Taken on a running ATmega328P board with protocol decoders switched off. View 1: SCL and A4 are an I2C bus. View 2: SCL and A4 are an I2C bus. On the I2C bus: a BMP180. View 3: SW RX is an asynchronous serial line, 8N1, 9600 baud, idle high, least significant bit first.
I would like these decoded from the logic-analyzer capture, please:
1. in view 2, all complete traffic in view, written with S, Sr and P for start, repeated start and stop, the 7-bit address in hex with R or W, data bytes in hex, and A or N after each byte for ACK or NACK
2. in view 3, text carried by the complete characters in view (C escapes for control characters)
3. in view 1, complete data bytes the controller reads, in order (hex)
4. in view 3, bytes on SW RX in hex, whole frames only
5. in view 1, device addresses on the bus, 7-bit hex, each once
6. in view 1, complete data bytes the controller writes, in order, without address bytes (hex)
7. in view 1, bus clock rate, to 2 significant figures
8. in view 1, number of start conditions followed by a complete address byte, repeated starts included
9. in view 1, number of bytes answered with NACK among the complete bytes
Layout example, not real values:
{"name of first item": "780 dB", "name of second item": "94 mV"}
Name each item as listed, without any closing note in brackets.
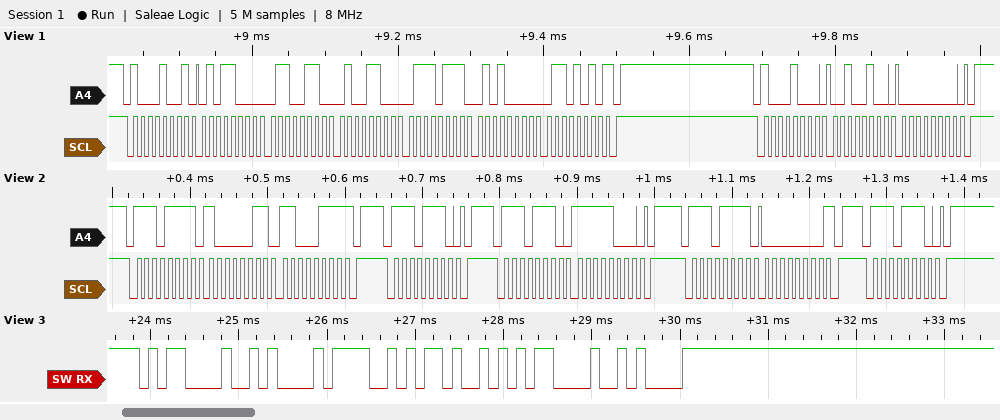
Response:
{"in view 2, all complete traffic in view, written with S, Sr and P for start, repeated start and stop, the 7-bit address in hex with R or W, data bytes in hex, and A or N after each byte for ACK or NACK": "S 77R A 83 A C7 N P S 77W A P S 77W A F8 A P S 77R A 00 N P S 77W A P", "in view 3, text carried by the complete characters in view": "\"\\r\\nOK\\r\\n\"", "in view 1, complete data bytes the controller reads, in order": "58 66 4C 77 50 6A", "in view 3, bytes on SW RX in hex, whole frames only": "0D 0A 4F 4B 0D 0A", "in view 1, device addresses on the bus, 7-bit hex, each once": "0x44", "in view 1, complete data bytes the controller writes, in order, without address bytes": "24 00", "in view 1, bus clock rate, to 2 significant figures": "100 kHz", "in view 1, number of start conditions followed by a complete address byte, repeated starts included": "2", "in view 1, number of bytes answered with NACK among the complete bytes": "1"}
